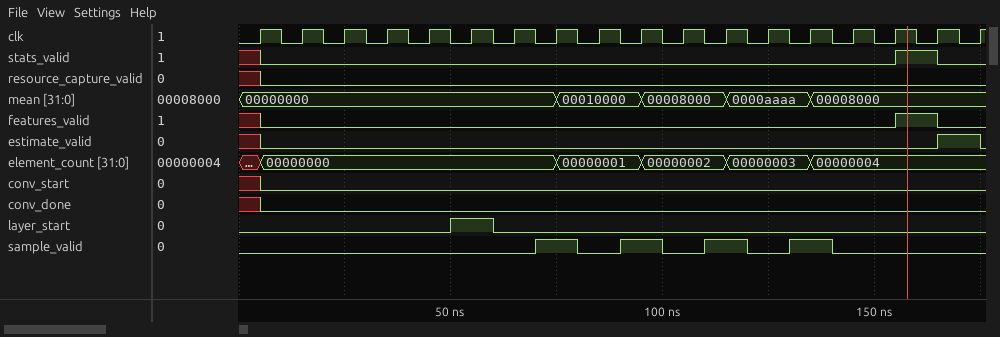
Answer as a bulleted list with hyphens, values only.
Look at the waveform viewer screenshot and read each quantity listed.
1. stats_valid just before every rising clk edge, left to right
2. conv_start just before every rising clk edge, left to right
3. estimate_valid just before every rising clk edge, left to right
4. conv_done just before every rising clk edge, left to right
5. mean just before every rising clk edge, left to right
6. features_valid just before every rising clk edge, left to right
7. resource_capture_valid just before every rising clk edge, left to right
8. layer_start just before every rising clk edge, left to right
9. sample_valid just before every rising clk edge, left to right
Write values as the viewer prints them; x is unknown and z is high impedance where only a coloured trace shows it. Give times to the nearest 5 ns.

- x 0 0 0 0 0 0 0 0 0 0 0 0 0 0 0 1 0
- x 0 0 0 0 0 0 0 0 0 0 0 0 0 0 0 0 0
- x 0 0 0 0 0 0 0 0 0 0 0 0 0 0 0 0 1
- x 0 0 0 0 0 0 0 0 0 0 0 0 0 0 0 0 0
- 00000000, 00000000, 00000000, 00000000, 00000000, 00000000, 00000000, 00000000, 00010000, 00010000, 00008000, 00008000, 0000aaaa, 0000aaaa, 00008000, 00008000, 00008000, 00008000
- x 0 0 0 0 0 0 0 0 0 0 0 0 0 0 0 1 0
- x 0 0 0 0 0 0 0 0 0 0 0 0 0 0 0 0 0
- 0 0 0 0 0 1 0 0 0 0 0 0 0 0 0 0 0 0
- 0 0 0 0 0 0 0 1 0 1 0 1 0 1 0 0 0 0
